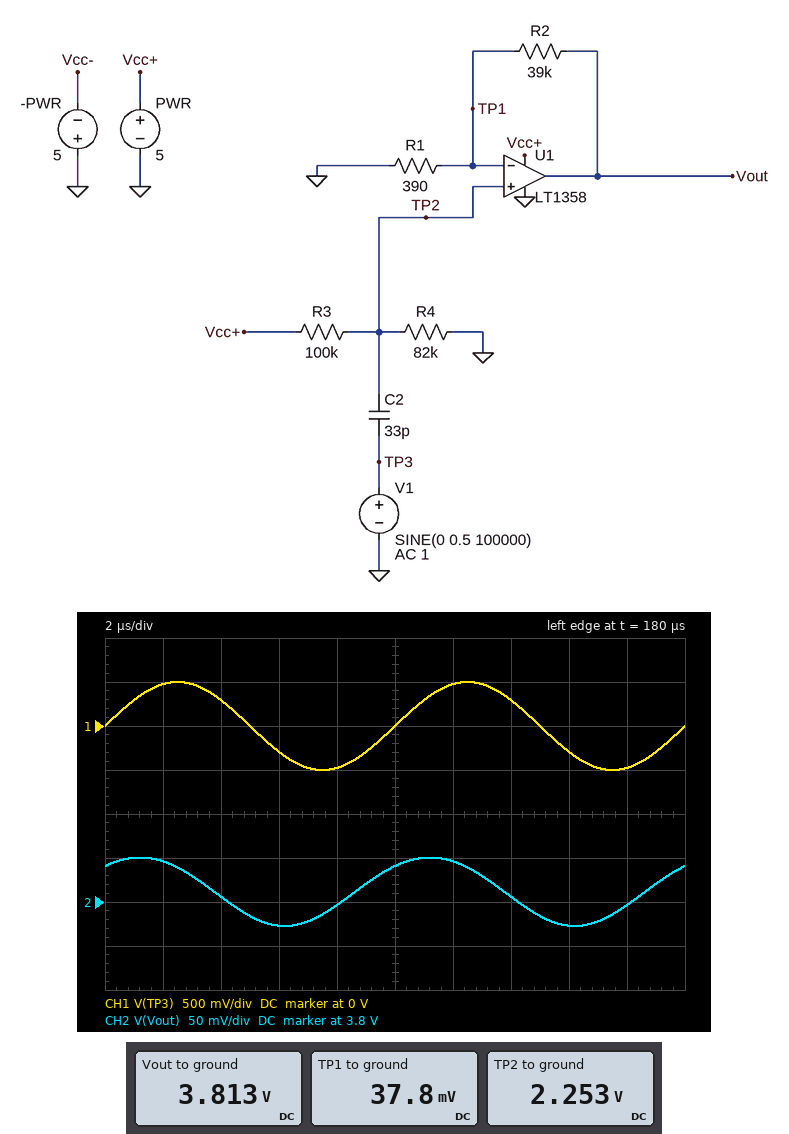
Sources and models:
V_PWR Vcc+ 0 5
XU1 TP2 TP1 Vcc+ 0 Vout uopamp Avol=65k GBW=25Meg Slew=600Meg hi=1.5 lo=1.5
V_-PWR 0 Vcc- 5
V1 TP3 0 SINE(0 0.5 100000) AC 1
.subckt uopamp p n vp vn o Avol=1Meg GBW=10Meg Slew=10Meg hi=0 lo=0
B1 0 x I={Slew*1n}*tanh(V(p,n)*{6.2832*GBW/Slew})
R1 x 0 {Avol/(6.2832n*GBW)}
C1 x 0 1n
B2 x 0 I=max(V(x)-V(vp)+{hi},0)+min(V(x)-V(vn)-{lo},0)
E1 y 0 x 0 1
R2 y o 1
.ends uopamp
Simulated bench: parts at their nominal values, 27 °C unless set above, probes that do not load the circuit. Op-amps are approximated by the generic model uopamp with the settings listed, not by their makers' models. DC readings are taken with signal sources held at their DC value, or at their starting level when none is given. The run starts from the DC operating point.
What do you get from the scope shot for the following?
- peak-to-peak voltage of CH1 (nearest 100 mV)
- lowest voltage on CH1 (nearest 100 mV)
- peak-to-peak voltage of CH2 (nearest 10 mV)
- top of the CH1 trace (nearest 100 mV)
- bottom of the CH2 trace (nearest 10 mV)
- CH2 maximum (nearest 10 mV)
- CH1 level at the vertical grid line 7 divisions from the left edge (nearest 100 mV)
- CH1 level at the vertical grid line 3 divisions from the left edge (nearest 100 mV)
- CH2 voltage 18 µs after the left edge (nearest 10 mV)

1.0 V
-500 mV
80 mV
500 mV
3.77 V
3.85 V
300 mV
-300 mV
3.80 V
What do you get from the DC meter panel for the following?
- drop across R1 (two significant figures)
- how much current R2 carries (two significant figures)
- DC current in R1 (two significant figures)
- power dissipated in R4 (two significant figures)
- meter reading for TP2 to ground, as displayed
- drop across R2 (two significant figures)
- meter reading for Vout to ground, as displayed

38 mV
97 µA
97 µA
62 µW
2.253 V
3.8 V
3.813 V
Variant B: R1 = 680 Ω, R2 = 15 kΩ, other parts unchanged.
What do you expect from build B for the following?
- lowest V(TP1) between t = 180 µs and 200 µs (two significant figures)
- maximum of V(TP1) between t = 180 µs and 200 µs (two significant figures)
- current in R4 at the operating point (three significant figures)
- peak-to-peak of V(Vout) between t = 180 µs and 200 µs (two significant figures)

160 mV
170 mV
27.5 µA
80 mV
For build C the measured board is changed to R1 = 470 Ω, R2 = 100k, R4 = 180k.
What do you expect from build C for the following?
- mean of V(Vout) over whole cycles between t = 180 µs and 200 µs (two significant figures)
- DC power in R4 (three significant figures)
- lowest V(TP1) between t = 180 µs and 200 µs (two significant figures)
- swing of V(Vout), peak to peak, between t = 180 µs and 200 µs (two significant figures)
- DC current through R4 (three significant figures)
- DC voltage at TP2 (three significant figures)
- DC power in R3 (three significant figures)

3.9 V
57.4 µW
18 mV
67 mV
17.9 µA
3.21 V
31.9 µW
